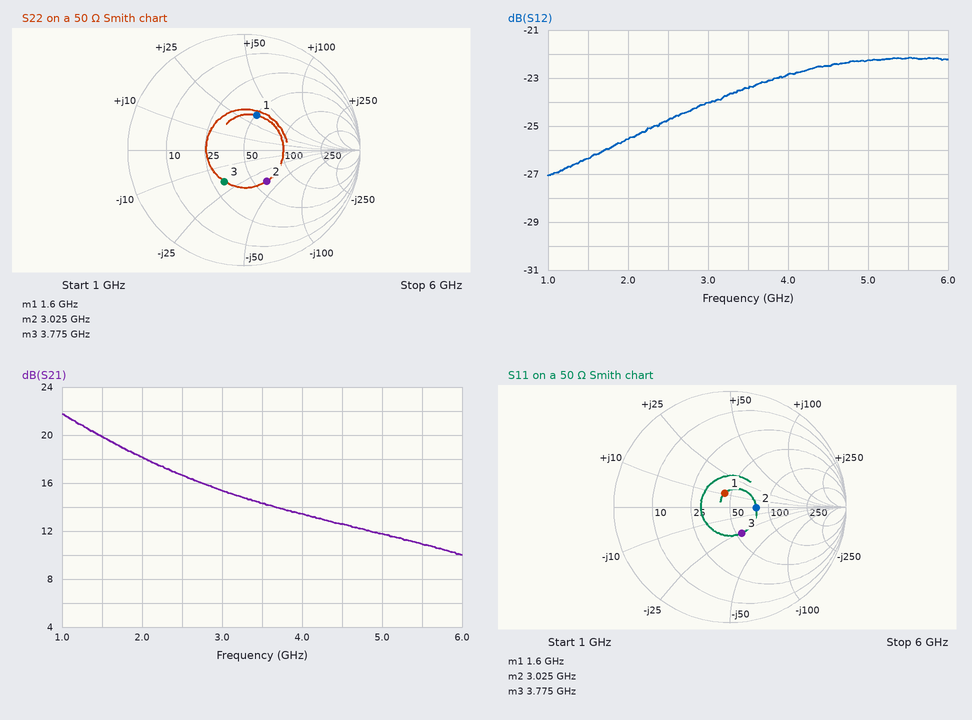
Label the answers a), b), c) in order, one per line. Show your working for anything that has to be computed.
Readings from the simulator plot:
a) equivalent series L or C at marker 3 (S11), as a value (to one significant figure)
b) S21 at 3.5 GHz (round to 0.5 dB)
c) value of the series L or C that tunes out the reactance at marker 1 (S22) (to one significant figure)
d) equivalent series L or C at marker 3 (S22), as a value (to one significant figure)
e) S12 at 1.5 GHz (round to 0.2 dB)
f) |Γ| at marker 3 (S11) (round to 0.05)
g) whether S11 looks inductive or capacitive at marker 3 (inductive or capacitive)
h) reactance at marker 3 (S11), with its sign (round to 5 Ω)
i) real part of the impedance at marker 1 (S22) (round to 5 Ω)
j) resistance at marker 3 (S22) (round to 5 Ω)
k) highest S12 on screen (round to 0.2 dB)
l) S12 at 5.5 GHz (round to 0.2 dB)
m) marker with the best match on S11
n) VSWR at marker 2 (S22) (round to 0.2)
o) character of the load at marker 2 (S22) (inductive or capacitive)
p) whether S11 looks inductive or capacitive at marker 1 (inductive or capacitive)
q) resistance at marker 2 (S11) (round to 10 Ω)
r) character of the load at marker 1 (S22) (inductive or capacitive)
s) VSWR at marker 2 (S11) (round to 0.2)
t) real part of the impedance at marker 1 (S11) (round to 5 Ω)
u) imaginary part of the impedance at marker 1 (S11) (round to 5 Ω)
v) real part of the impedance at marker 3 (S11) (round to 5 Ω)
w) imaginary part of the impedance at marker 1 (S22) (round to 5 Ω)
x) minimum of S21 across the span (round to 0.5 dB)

a) C = 1/(2π × 3.775 GHz × 25 Ω) ≈ 2 pF
b) 14.5 dB
c) C = 1/(2π × 1.6 GHz × 35 Ω) ≈ 3 pF
d) C = 1/(2π × 3.775 GHz × 20 Ω) ≈ 2 pF
e) -26.4 dB
f) 0.25
g) capacitive
h) -25 Ω
i) 50 Ω
j) 30 Ω
k) -22.2 dB
l) -22.2 dB
m) marker 1
n) 2.0
o) capacitive
p) inductive
q) 80 Ω
r) inductive
s) 1.6
t) 45 Ω
u) +10 Ω
v) 55 Ω
w) +35 Ω
x) 10.0 dB
